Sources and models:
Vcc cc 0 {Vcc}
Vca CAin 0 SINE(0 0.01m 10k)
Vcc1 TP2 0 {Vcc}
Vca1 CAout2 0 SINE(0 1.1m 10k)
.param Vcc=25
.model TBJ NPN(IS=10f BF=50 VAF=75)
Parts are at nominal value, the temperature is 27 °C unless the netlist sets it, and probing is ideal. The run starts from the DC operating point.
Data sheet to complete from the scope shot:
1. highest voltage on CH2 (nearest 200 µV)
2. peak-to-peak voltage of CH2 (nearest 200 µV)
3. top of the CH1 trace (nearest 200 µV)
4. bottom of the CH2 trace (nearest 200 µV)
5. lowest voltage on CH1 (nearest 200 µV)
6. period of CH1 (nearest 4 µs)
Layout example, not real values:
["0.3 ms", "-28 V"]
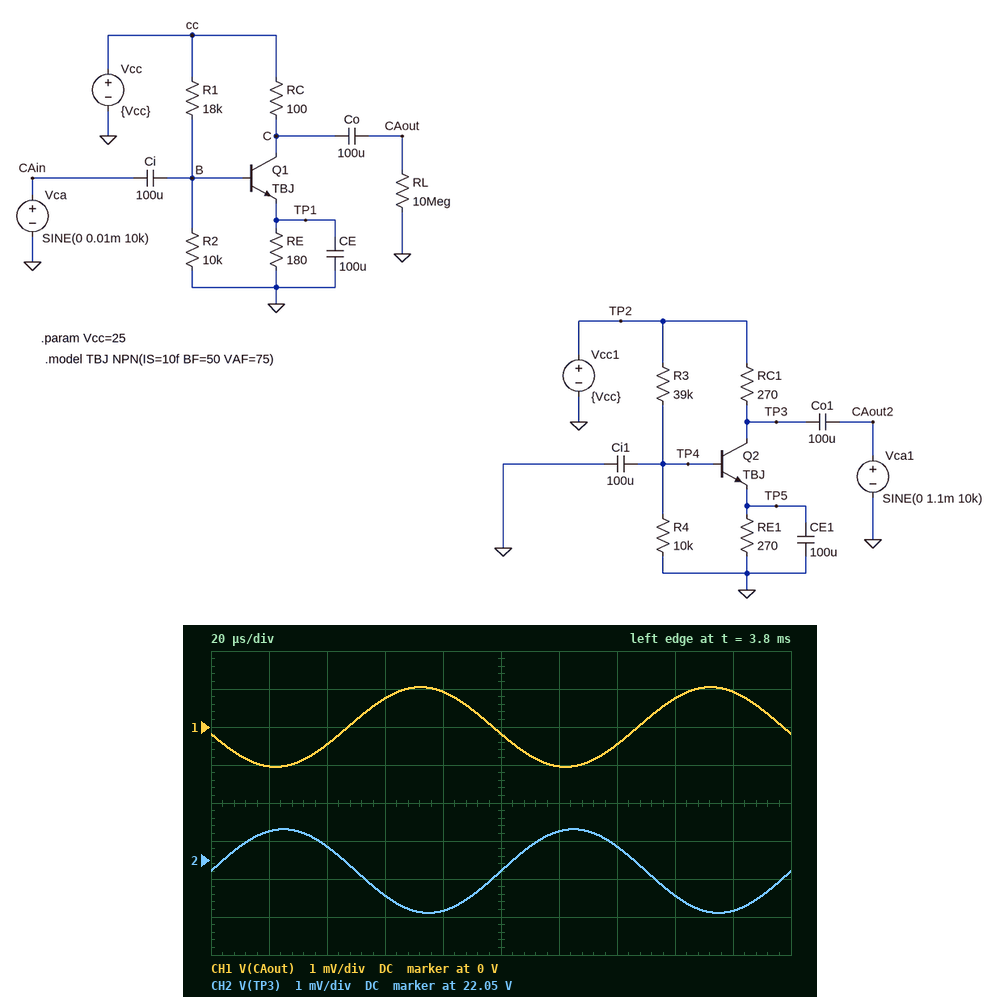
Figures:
["22.0538 V", "2.2 mV", "1.0 mV", "22.0516 V", "-1.0 mV", "100 µs"]
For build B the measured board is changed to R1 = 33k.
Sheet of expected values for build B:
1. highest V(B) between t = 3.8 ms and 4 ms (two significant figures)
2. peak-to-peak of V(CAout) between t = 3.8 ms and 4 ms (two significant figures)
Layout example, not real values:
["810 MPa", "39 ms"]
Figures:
["3.8 V", "1.3 mV"]
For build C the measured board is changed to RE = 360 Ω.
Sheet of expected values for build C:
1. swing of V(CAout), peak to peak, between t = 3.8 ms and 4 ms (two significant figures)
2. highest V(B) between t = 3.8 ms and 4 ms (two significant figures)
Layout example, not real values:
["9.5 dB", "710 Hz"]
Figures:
["1.3 mV", "7.1 V"]
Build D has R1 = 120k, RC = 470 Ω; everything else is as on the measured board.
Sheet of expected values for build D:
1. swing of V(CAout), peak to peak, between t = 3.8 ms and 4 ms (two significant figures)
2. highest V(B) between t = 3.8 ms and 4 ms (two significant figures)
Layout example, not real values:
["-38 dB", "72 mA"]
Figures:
["1.4 mV", "1.4 V"]
